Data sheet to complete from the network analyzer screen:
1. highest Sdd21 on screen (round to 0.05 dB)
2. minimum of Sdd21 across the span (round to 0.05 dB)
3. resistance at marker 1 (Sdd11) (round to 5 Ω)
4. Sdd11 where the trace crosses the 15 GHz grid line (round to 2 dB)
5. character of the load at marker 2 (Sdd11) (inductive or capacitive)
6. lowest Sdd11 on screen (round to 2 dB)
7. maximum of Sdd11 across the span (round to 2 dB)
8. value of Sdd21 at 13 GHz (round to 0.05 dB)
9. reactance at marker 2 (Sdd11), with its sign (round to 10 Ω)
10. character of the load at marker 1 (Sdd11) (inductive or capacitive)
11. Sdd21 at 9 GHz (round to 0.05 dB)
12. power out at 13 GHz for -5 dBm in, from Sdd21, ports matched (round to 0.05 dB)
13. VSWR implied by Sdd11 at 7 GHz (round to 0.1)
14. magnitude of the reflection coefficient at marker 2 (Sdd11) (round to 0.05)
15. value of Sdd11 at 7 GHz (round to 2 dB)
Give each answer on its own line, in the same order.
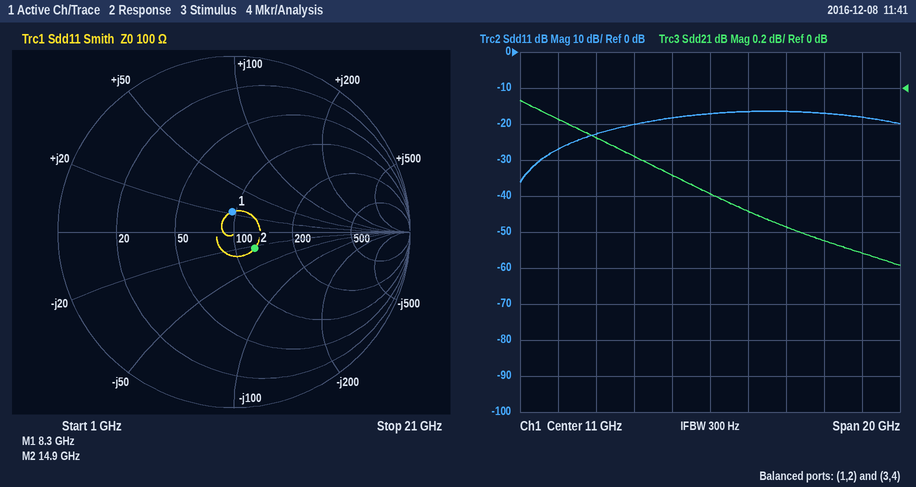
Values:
-0.05 dB
-1.00 dB
95 Ω
-16 dB
capacitive
-36 dB
-16 dB
-0.70 dB
-20 Ω
inductive
-0.50 dB
-5.70 dBm
1.2
0.15
-20 dB
